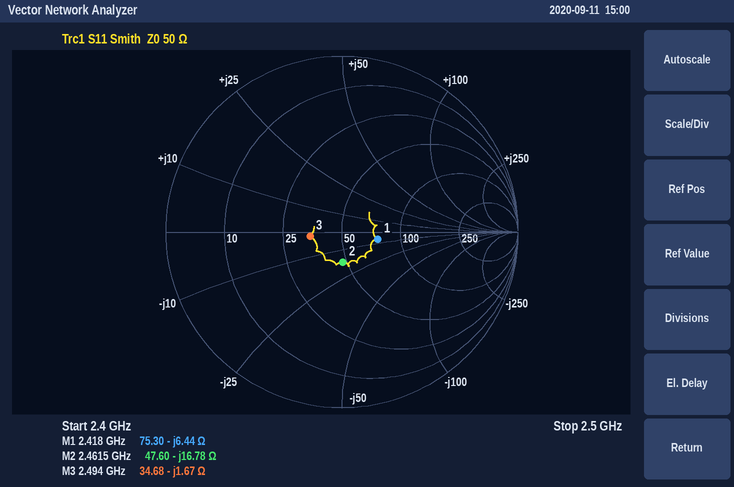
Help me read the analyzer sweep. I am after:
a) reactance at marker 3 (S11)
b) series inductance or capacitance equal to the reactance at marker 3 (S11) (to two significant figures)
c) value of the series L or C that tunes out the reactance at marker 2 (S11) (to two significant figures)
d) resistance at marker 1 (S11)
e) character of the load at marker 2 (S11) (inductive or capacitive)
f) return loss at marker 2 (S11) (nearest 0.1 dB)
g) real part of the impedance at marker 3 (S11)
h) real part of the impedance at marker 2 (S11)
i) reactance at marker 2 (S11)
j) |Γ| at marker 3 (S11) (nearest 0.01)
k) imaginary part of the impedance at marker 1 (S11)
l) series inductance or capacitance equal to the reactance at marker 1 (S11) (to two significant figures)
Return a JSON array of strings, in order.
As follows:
["-1.67 Ω", "38 pF", "1.1 nH", "75.30 Ω", "capacitive", "15.3 dB", "34.68 Ω", "47.60 Ω", "-16.78 Ω", "0.18", "-6.44 Ω", "10 pF"]
